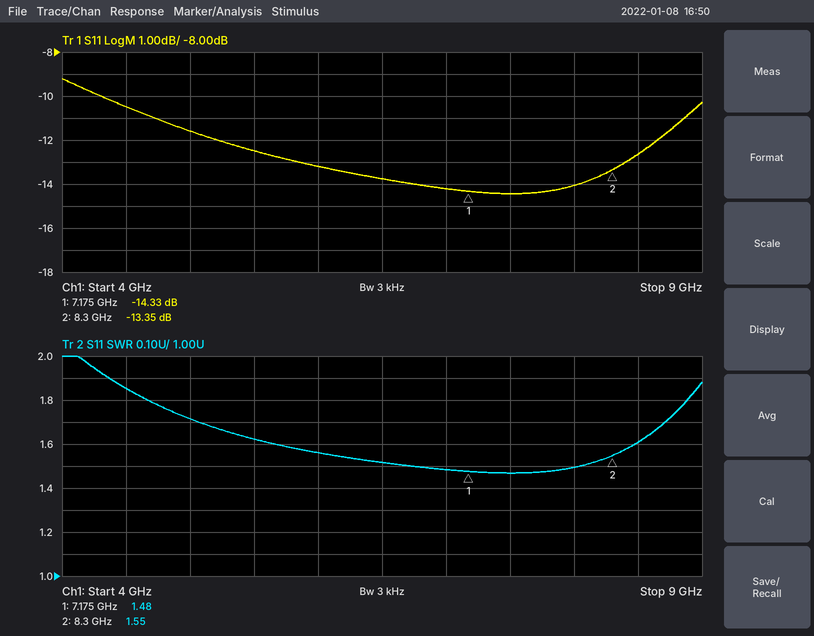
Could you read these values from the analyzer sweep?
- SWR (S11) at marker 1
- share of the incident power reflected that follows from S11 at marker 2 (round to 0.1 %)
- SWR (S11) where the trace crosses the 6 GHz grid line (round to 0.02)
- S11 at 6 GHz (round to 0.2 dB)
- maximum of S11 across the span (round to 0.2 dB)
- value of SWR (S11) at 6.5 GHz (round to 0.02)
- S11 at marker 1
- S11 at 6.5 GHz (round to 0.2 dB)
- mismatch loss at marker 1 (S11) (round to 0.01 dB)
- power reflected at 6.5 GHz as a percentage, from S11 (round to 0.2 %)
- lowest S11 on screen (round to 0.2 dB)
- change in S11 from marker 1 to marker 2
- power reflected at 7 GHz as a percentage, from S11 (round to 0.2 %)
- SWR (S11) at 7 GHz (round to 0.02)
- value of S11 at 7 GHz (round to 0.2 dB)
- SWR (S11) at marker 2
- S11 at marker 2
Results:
1.48
4.6 %
1.56
-13.2 dB
-9.2 dB
1.52
-14.33 dB
-13.8 dB
0.16 dB
4.2 %
-14.4 dB
0.98 dB
3.8 %
1.48
-14.2 dB
1.55
-13.35 dB
